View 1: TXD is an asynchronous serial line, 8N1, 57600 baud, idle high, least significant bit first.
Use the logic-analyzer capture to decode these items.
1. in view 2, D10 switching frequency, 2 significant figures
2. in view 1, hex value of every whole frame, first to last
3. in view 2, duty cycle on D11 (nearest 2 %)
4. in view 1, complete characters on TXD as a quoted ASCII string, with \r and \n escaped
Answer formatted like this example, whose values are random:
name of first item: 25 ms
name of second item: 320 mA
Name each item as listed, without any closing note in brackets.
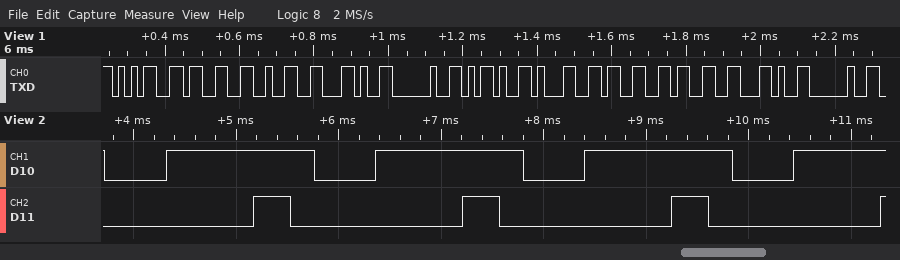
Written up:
in view 2, D10 switching frequency, 2 significant figures: 490 Hz
in view 1, hex value of every whole frame, first to last: 35 33 32 2C 20 2D 31 33 33 2C 20
in view 2, duty cycle on D11: 18 %
in view 1, complete characters on TXD as a quoted ASCII string, with \r and \n escaped: "532, -133, "
